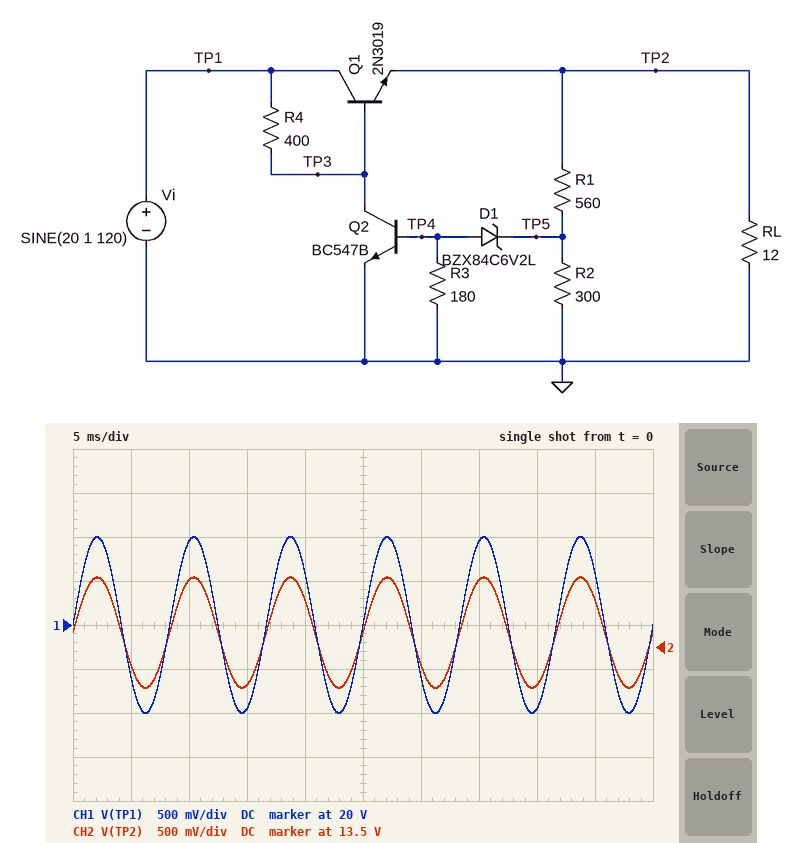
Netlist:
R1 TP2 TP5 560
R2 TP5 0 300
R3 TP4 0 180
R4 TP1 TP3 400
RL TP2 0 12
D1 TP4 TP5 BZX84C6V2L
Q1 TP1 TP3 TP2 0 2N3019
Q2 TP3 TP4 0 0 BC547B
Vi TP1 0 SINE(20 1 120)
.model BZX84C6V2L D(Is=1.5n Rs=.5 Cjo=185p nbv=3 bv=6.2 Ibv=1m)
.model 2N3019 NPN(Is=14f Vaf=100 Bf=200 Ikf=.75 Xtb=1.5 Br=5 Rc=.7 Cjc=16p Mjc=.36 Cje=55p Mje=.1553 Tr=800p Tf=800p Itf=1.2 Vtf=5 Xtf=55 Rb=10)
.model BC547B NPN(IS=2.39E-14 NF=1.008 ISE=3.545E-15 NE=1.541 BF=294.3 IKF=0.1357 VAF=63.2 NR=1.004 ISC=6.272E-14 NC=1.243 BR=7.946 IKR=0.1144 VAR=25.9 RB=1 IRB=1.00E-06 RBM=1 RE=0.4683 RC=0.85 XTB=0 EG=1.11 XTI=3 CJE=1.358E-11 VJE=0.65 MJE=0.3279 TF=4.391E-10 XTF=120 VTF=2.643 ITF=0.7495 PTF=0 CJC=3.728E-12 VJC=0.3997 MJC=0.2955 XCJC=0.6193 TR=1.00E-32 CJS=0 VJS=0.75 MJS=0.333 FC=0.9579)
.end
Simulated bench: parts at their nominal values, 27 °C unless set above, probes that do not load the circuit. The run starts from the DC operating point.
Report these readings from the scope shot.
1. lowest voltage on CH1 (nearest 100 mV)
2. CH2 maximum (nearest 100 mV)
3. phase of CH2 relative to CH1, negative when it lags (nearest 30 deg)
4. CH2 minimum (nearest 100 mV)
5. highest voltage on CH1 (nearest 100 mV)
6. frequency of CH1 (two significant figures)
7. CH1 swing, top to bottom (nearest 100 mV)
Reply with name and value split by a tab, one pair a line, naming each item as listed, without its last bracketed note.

lowest voltage on CH1	19.0 V
CH2 maximum	14.3 V
phase of CH2 relative to CH1, negative when it lags	0 deg
CH2 minimum	13.0 V
highest voltage on CH1	21.0 V
frequency of CH1	120 Hz
CH1 swing, top to bottom	2.0 V
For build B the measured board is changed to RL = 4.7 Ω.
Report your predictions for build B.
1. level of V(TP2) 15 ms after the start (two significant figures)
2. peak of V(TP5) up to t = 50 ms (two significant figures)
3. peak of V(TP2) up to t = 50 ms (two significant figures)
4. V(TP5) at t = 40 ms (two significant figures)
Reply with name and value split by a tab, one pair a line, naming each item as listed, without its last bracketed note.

level of V(TP2) 15 ms after the start	8.1 V
peak of V(TP5) up to t = 50 ms	3.1 V
peak of V(TP2) up to t = 50 ms	8.8 V
V(TP5) at t = 40 ms	2.8 V
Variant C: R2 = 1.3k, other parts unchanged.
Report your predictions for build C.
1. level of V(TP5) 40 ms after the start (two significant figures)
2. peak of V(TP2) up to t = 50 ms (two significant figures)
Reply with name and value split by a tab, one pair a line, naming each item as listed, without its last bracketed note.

level of V(TP5) 40 ms after the start	7.0 V
peak of V(TP2) up to t = 50 ms	12 V
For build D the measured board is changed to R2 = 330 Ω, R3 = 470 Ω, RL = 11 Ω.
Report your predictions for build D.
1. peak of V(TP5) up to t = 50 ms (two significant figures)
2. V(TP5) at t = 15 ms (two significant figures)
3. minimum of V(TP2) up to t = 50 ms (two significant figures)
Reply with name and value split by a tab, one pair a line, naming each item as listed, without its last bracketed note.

peak of V(TP5) up to t = 50 ms	5.1 V
V(TP5) at t = 15 ms	4.7 V
minimum of V(TP2) up to t = 50 ms	13 V
